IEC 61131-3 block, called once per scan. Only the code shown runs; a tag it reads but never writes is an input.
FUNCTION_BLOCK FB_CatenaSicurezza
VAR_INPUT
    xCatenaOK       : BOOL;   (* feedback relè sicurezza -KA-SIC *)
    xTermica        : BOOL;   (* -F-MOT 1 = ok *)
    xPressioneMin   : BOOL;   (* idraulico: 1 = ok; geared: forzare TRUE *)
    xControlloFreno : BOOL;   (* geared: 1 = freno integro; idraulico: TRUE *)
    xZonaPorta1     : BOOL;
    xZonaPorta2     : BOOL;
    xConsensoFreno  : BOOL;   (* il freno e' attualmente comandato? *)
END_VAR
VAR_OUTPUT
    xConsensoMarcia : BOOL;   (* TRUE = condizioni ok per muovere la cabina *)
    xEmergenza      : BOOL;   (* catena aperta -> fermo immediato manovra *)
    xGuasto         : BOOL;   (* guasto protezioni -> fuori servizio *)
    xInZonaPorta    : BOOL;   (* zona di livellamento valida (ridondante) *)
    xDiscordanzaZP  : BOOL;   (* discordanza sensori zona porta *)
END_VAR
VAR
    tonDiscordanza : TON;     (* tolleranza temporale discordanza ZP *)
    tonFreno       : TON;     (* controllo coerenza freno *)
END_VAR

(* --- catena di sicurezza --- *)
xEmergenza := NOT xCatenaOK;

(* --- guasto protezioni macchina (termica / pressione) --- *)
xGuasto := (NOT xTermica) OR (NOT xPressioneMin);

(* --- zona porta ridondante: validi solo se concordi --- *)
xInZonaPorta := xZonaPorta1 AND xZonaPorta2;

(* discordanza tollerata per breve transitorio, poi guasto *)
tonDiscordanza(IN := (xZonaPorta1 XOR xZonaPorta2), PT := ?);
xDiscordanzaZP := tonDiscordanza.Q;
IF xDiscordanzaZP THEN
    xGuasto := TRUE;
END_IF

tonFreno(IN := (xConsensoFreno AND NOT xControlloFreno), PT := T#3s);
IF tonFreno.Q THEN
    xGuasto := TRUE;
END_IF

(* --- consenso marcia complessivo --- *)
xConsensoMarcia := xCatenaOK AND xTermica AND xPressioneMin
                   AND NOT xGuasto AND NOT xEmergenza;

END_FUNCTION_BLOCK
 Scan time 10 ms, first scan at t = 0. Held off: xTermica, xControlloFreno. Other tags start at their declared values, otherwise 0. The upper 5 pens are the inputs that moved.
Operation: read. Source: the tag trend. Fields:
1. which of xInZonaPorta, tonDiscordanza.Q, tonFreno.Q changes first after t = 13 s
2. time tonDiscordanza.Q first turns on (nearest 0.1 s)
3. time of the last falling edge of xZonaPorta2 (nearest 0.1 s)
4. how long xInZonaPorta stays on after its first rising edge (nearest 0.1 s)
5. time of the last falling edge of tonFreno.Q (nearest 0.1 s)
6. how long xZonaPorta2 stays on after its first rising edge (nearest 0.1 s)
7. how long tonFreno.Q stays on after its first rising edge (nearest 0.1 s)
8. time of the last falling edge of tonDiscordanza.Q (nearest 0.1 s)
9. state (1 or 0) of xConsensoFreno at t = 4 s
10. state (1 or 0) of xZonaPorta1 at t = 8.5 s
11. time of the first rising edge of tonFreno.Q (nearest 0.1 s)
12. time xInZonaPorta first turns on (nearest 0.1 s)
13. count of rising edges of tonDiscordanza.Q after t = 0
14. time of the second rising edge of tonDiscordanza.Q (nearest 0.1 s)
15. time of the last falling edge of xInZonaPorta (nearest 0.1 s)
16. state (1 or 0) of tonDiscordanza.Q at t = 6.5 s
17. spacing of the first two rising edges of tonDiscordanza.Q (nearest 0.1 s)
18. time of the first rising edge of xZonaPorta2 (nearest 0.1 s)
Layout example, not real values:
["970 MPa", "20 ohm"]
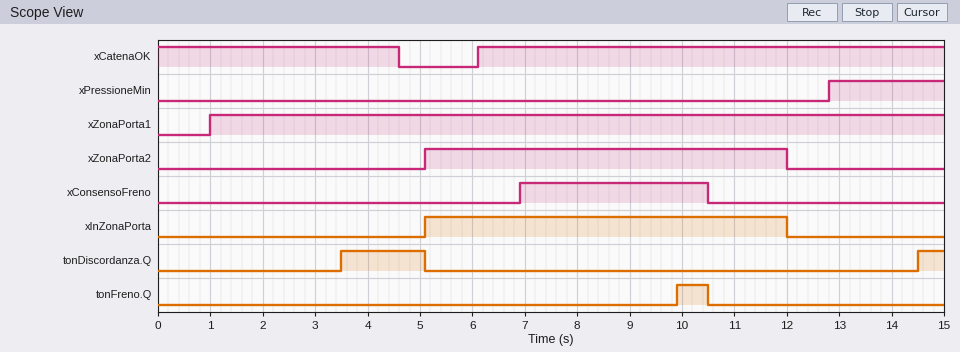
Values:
["tonDiscordanza.Q", "3.5 s", "12.0 s", "6.9 s", "10.5 s", "6.9 s", "0.6 s", "5.1 s", "0", "1", "9.9 s", "5.1 s", "2", "14.5 s", "12.0 s", "0", "11.0 s", "5.1 s"]
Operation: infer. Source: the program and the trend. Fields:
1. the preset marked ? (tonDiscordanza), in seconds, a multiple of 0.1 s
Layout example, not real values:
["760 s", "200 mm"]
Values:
["2.5 s"]
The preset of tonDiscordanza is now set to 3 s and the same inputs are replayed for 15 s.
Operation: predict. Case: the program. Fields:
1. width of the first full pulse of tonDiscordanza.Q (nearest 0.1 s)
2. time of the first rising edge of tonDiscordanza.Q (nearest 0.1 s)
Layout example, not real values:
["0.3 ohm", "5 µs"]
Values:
["1.1 s", "4.0 s"]
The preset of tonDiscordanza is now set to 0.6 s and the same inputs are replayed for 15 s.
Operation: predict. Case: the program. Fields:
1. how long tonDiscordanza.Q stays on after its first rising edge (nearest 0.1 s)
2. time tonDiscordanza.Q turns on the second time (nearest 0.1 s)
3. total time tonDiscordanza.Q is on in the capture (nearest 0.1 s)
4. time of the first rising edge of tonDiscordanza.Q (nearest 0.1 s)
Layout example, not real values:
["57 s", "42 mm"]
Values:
["3.5 s", "12.6 s", "5.9 s", "1.6 s"]
